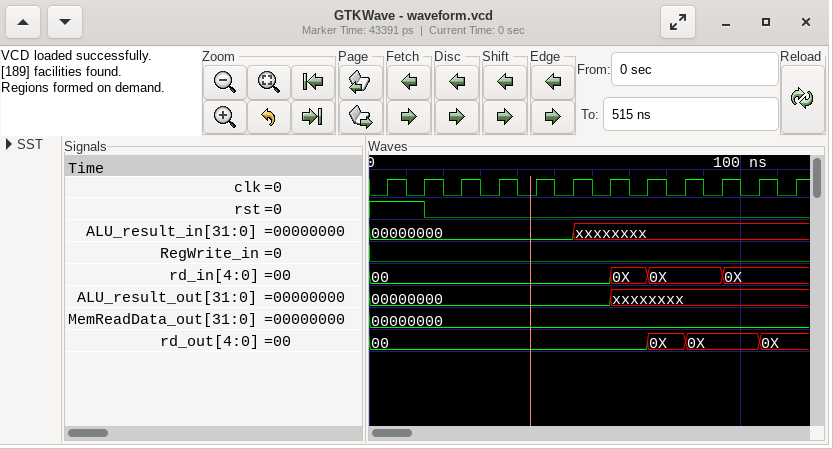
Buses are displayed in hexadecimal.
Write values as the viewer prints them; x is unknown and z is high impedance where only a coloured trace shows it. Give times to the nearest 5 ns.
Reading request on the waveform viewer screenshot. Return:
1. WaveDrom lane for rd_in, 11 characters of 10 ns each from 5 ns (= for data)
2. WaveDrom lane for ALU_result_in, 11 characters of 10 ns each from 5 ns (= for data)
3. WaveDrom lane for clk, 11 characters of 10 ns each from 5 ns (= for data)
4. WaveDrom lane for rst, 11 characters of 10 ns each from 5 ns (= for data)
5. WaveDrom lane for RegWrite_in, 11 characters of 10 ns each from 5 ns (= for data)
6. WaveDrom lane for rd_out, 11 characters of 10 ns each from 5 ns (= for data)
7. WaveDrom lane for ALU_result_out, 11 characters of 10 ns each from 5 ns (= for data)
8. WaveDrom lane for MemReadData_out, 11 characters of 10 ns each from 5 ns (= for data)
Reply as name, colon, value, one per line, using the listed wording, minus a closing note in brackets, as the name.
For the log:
WaveDrom lane for rd_in, 11 characters of 10 ns each from 5 ns: {name: 'rd_in', wave: '=.....==.=.', data: '00 0X 0X 0X'}
WaveDrom lane for ALU_result_in, 11 characters of 10 ns each from 5 ns: {name: 'ALU_result_in', wave: '=....x.....', data: '00000000'}
WaveDrom lane for clk, 11 characters of 10 ns each from 5 ns: {name: 'clk', wave: 'p..........'}
WaveDrom lane for rst, 11 characters of 10 ns each from 5 ns: {name: 'rst', wave: '10.........'}
WaveDrom lane for RegWrite_in, 11 characters of 10 ns each from 5 ns: {name: 'RegWrite_in', wave: '0..........'}
WaveDrom lane for rd_out, 11 characters of 10 ns each from 5 ns: {name: 'rd_out', wave: '=......==.=', data: '00 0X 0X 0X'}
WaveDrom lane for ALU_result_out, 11 characters of 10 ns each from 5 ns: {name: 'ALU_result_out', wave: '=.....x....', data: '00000000'}
WaveDrom lane for MemReadData_out, 11 characters of 10 ns each from 5 ns: {name: 'MemReadData_out', wave: '=..........', data: '00000000'}
